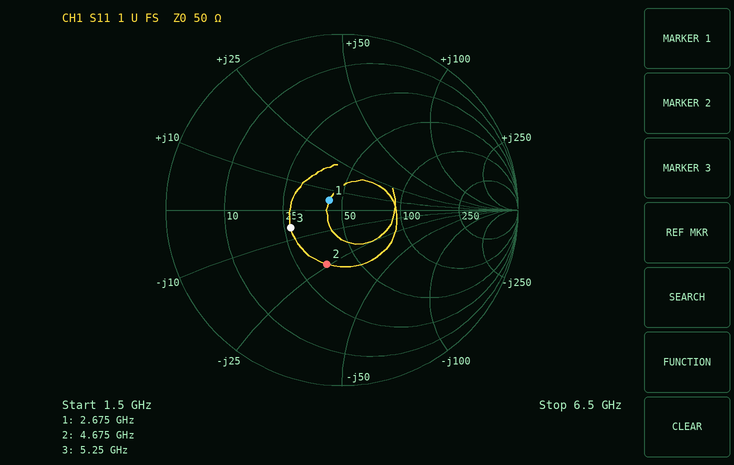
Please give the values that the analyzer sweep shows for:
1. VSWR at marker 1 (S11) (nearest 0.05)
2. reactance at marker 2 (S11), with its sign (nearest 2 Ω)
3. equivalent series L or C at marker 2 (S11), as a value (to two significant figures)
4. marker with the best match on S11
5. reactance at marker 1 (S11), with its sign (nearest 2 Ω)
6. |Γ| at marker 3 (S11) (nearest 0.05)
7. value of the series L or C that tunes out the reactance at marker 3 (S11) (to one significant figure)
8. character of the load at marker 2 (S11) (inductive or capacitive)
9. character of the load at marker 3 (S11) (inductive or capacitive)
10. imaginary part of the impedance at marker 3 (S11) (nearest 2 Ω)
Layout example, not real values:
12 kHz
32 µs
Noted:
1.20
-24 Ω
1.4 pF
marker 1
+4 Ω
0.30
200 pH
capacitive
capacitive
-6 Ω
